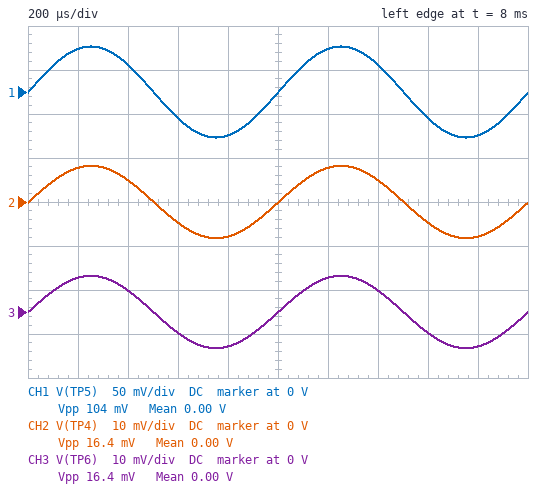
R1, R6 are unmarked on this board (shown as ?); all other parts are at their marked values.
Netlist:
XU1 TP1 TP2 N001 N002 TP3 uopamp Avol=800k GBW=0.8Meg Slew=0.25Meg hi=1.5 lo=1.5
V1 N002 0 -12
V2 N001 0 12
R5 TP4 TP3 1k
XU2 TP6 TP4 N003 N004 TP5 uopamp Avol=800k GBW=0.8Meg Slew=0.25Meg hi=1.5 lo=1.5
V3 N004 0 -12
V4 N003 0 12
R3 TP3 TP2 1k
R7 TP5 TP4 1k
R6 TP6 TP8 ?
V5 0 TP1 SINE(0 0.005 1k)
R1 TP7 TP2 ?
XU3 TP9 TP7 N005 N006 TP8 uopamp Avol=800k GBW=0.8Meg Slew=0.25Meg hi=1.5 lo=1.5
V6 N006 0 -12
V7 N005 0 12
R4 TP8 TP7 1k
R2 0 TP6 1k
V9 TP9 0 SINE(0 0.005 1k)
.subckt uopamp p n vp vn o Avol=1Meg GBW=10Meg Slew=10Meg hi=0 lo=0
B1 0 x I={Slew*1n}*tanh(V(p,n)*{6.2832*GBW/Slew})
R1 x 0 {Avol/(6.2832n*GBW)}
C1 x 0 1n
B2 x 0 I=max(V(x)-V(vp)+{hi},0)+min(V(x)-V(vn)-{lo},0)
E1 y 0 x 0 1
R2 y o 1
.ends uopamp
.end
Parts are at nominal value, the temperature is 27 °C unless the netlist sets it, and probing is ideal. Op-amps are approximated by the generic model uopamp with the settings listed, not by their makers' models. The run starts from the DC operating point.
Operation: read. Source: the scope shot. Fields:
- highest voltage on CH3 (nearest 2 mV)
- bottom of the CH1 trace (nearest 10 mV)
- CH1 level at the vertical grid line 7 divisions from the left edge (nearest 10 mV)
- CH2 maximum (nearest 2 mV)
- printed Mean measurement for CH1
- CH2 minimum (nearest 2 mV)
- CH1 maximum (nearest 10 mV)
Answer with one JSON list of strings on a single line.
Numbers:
["8 mV", "-50 mV", "30 mV", "8 mV", "0.00 V", "-8 mV", "50 mV"]
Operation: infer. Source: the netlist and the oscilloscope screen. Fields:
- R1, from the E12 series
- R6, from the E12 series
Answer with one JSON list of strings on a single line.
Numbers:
["330 Ω", "3.3 kΩ"]
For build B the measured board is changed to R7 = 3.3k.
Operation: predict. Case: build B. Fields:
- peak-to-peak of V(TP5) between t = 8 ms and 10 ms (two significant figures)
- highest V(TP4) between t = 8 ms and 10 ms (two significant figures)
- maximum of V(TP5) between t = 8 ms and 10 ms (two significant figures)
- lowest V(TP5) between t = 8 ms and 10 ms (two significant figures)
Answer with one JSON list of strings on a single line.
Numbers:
["300 mV", "8.2 mV", "150 mV", "-150 mV"]
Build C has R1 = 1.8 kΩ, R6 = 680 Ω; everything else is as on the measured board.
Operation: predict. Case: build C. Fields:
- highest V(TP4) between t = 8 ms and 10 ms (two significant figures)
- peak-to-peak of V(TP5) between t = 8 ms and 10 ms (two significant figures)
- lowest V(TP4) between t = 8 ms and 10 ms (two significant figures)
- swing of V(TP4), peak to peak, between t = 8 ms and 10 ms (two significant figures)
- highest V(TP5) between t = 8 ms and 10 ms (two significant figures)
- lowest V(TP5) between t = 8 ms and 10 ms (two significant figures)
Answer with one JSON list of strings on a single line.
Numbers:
["6.3 mV", "46 mV", "-6.3 mV", "13 mV", "23 mV", "-23 mV"]
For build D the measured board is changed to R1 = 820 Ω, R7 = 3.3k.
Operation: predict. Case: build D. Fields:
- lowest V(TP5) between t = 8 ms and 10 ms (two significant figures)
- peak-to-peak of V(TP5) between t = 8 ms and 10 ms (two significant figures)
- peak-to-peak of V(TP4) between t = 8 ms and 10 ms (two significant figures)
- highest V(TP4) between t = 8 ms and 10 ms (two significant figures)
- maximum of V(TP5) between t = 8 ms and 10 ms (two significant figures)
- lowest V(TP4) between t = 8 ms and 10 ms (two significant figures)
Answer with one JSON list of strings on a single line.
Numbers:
["-74 mV", "150 mV", "8.0 mV", "4.0 mV", "74 mV", "-4.0 mV"]
